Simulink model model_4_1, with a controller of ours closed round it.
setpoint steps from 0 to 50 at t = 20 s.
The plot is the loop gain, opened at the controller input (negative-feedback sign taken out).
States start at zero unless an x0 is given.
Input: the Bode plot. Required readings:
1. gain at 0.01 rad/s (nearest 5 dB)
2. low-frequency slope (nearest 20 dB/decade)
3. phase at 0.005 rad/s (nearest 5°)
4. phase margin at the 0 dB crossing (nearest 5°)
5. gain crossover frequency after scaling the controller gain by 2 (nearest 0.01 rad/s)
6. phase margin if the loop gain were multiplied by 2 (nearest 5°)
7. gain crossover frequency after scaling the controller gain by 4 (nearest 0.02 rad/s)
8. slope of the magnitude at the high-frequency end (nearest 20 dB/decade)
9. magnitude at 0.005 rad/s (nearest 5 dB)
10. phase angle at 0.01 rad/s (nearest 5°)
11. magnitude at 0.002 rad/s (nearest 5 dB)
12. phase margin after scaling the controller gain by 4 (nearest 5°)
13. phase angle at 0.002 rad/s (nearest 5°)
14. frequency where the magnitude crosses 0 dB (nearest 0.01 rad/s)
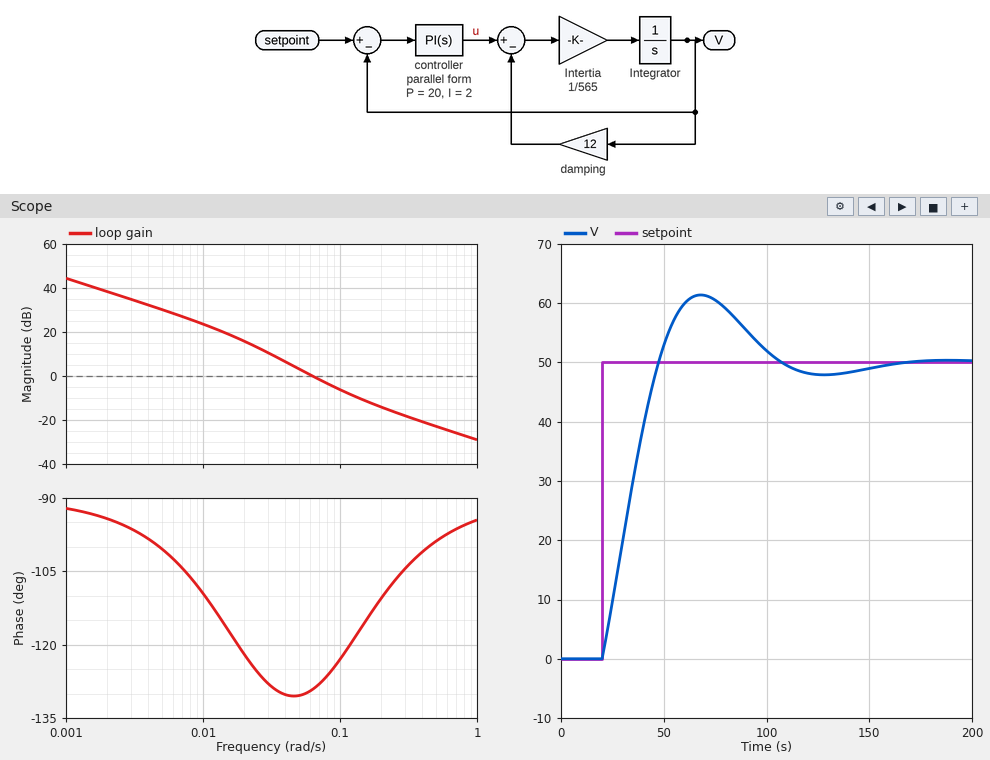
25 dB
-20 dB/decade
-100°
50°
0.10 rad/s
55°
0.16 rad/s
-20 dB/decade
30 dB
-110°
40 dB
65°
-95°
0.06 rad/s
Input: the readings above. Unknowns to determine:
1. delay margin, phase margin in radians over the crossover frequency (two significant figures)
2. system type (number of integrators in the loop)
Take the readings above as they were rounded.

15 s
1
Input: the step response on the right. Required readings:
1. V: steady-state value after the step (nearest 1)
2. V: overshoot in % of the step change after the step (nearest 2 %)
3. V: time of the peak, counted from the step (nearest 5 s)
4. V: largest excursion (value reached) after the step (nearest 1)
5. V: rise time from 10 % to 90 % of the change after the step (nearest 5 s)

50
22 %
50 s
61
20 s
